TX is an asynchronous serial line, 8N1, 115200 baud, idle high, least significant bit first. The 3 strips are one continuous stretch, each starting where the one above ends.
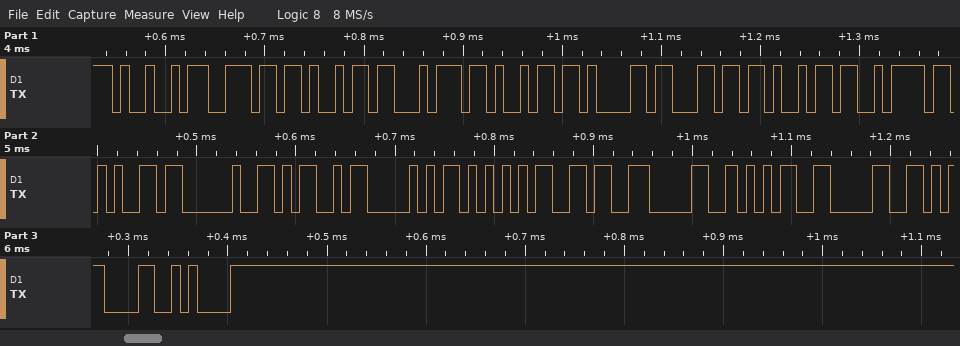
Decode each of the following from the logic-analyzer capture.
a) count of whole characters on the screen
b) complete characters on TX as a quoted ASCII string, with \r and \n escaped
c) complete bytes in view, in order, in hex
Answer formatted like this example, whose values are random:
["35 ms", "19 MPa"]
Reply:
["20", "\"Initialize MPU6050\\r\\n\"", "0x49 0x6E 0x69 0x74 0x69 0x61 0x6C 0x69 0x7A 0x65 0x20 0x4D 0x50 0x55 0x36 0x30 0x35 0x30 0x0D 0x0A"]
